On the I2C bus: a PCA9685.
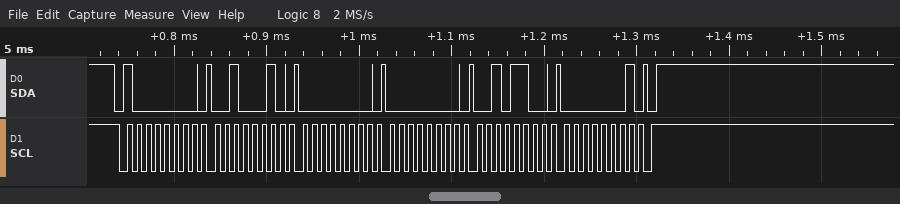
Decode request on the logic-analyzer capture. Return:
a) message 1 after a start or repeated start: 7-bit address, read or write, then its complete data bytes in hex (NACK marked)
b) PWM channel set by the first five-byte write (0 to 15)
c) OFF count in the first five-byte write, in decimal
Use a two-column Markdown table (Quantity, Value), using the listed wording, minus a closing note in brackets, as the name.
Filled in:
| Quantity | Value |
|---|---|
| message 1 after a start or repeated start: 7-bit address, read or write, then its complete data bytes in hex | 0x40 write: 22 00 00 2C 01 |
| PWM channel set by the first five-byte write | 7 |
| OFF count in the first five-byte write, in decimal | 300 |
